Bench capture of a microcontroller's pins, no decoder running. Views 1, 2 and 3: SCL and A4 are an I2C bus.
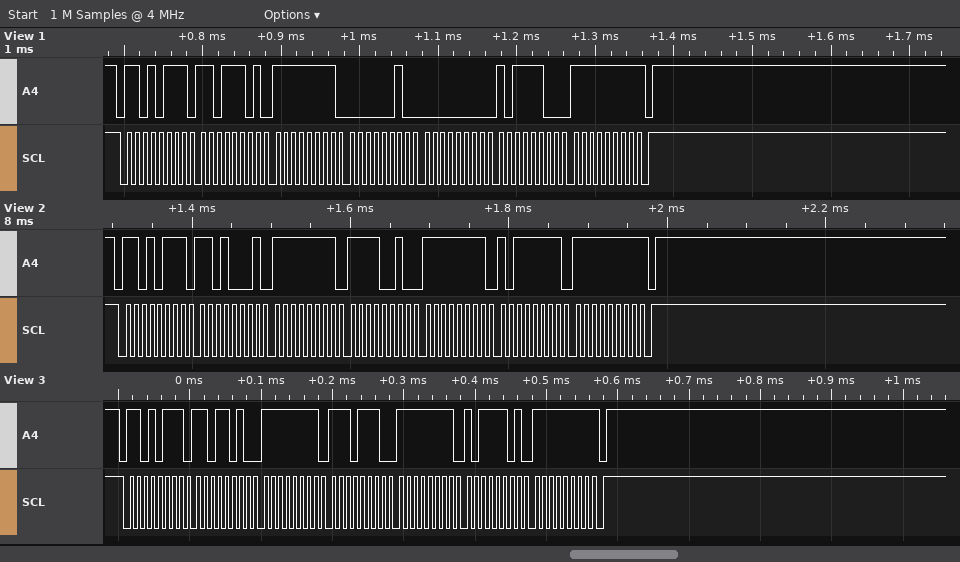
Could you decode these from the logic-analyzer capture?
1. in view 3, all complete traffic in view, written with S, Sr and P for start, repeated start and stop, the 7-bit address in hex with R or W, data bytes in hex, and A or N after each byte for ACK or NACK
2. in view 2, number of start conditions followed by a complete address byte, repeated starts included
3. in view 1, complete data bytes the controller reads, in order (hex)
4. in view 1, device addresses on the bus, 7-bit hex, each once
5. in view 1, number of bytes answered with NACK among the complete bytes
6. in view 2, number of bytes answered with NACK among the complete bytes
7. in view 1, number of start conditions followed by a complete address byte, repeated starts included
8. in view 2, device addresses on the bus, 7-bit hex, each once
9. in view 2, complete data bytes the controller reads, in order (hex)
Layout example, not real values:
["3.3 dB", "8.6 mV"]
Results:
["S 6BR A DA A FF A EE A FF A BD A FF N P", "1", "DD FF 02 00 BC FF", "0x6B", "1", "1", "1", "0x6B", "D1 FF F2 FF BF FF"]
